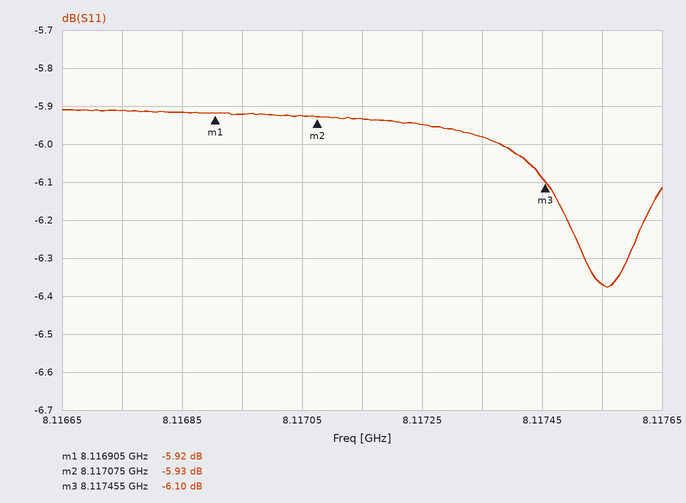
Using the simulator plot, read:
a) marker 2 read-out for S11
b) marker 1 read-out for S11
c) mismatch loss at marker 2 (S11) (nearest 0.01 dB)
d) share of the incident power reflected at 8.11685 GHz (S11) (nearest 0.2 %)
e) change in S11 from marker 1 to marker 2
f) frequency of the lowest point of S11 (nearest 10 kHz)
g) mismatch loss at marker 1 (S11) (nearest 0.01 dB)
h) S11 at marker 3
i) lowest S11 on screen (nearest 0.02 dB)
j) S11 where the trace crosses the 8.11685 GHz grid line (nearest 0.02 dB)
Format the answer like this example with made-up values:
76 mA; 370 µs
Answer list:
-5.93 dB; -5.92 dB; 1.28 dB; 25.6 %; -0.01 dB; 8.11756 GHz; 1.28 dB; -6.10 dB; -6.38 dB; -5.92 dB
